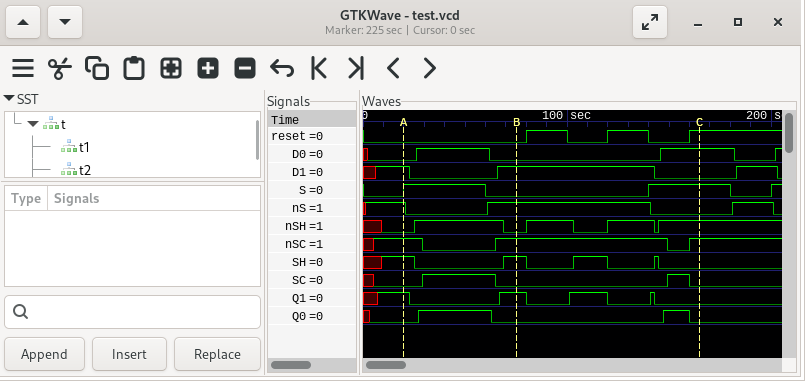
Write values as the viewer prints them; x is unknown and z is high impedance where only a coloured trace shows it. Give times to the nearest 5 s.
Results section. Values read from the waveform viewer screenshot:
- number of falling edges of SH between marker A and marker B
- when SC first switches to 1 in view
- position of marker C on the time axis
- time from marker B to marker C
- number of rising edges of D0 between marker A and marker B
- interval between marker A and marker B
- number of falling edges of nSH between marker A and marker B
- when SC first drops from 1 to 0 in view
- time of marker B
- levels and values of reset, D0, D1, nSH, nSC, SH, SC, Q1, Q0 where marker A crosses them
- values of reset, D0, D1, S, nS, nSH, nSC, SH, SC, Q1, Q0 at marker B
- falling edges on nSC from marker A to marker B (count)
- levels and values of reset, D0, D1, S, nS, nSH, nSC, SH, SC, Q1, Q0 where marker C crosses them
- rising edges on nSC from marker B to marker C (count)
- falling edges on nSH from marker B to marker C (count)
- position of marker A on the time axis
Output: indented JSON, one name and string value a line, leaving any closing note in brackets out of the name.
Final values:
{
  "number of falling edges of SH between marker A and marker B": "1",
  "when SC first switches to 1 in view": "30 s",
  "position of marker C on the time axis": "165 s",
  "time from marker B to marker C": "90 s",
  "number of rising edges of D0 between marker A and marker B": "1",
  "interval between marker A and marker B": "55 s",
  "number of falling edges of nSH between marker A and marker B": "1",
  "when SC first drops from 1 to 0 in view": "65 s",
  "time of marker B": "75 s",
  "levels and values of reset, D0, D1, nSH, nSC, SH, SC, Q1, Q0 where marker A crosses them": "reset=0, D0=0, D1=1, nSH=0, nSC=1, SH=1, SC=0, Q1=1, Q0=0",
  "values of reset, D0, D1, S, nS, nSH, nSC, SH, SC, Q1, Q0 at marker B": "reset=0, D0=0, D1=1, S=0, nS=1, nSH=0, nSC=1, SH=1, SC=0, Q1=1, Q0=0",
  "falling edges on nSC from marker A to marker B": "1",
  "levels and values of reset, D0, D1, S, nS, nSH, nSC, SH, SC, Q1, Q0 where marker C crosses them": "reset=1, D0=1, D1=0, S=1, nS=0, nSH=1, nSC=1, SH=0, SC=0, Q1=0, Q0=0",
  "rising edges on nSC from marker B to marker C": "1",
  "falling edges on nSH from marker B to marker C": "2",
  "position of marker A on the time axis": "20 s"
}
